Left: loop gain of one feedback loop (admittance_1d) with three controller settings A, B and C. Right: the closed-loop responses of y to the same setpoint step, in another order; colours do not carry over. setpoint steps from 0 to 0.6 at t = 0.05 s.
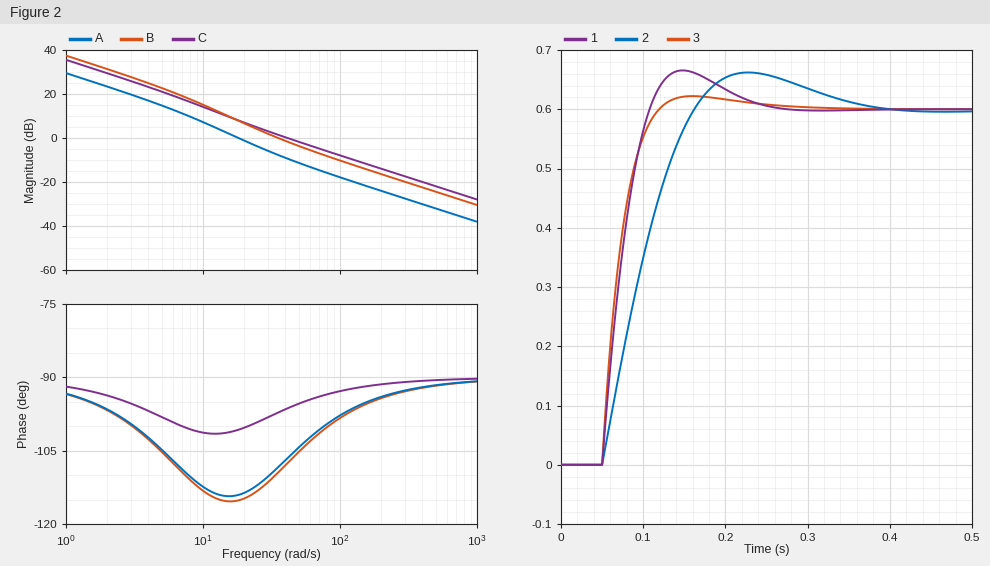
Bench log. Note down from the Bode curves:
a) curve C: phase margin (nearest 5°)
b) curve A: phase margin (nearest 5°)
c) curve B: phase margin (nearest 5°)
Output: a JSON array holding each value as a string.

["85°", "65°", "70°"]
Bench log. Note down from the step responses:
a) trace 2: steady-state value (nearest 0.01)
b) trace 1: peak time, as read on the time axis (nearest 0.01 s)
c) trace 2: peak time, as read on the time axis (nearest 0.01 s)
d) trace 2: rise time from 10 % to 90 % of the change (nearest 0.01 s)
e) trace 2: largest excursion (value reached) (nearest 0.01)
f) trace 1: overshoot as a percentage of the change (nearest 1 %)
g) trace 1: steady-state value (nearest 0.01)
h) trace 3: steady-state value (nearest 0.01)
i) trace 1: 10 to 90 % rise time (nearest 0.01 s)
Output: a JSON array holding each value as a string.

["0.60", "0.15 s", "0.23 s", "0.08 s", "0.66", "11 %", "0.60", "0.60", "0.04 s"]
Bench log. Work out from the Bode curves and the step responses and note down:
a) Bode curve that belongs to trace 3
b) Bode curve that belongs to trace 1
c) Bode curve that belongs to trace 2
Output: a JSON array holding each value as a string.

["C", "B", "A"]
